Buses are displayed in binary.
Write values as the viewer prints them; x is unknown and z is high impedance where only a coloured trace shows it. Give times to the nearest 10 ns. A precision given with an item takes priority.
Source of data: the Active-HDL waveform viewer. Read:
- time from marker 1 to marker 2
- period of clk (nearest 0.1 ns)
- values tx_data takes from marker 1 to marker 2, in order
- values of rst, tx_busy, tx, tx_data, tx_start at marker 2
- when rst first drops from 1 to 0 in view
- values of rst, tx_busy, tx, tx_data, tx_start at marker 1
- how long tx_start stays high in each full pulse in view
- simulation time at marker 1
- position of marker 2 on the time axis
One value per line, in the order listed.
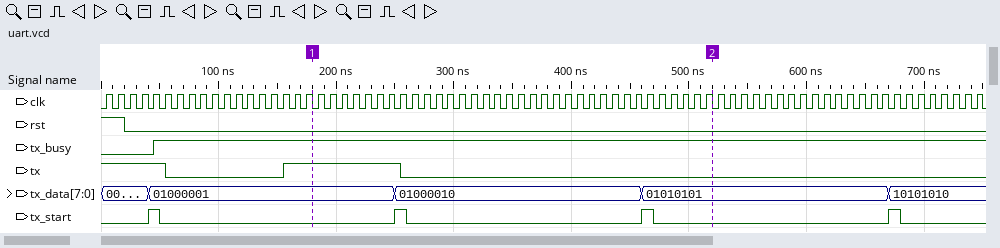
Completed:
340 ns
10 ns
01000001, 01000010, 01010101
rst=0, tx_busy=1, tx=0, tx_data=01010101, tx_start=0
20 ns
rst=0, tx_busy=1, tx=1, tx_data=01000001, tx_start=0
10 ns, 10 ns, 10 ns, 10 ns
180 ns
520 ns
